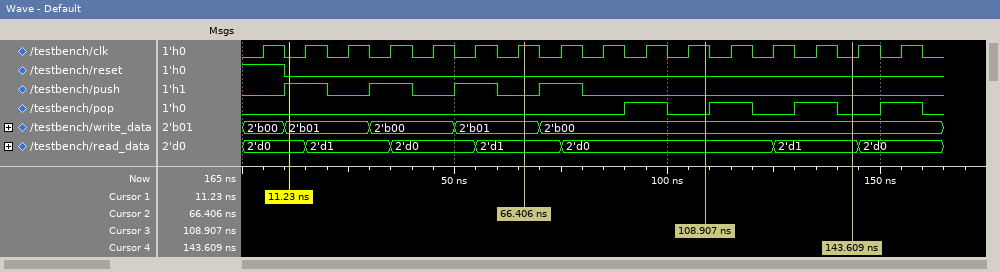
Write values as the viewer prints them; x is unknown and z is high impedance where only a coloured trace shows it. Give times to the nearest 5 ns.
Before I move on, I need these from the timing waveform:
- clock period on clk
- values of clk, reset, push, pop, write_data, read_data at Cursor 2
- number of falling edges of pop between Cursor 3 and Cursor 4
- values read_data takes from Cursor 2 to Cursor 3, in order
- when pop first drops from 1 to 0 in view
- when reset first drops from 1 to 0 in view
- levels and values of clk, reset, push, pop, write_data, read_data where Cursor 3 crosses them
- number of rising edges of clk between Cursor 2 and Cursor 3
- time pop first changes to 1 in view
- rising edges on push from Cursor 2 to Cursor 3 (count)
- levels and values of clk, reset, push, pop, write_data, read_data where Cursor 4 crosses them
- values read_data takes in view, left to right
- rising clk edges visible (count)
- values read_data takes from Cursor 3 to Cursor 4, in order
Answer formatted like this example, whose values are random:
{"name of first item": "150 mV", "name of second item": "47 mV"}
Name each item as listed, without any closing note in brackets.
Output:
{"clock period on clk": "10 ns", "values of clk, reset, push, pop, write_data, read_data at Cursor 2": "clk=1, reset=0, push=0, pop=0, write_data=2'b01, read_data=2'd1", "number of falling edges of pop between Cursor 3 and Cursor 4": "2", "values read_data takes from Cursor 2 to Cursor 3, in order": "2'd1, 2'd0", "when pop first drops from 1 to 0 in view": "100 ns", "when reset first drops from 1 to 0 in view": "10 ns", "levels and values of clk, reset, push, pop, write_data, read_data where Cursor 3 crosses them": "clk=1, reset=0, push=0, pop=0, write_data=2'b00, read_data=2'd0", "number of rising edges of clk between Cursor 2 and Cursor 3": "4", "time pop first changes to 1 in view": "90 ns", "rising edges on push from Cursor 2 to Cursor 3": "1", "levels and values of clk, reset, push, pop, write_data, read_data where Cursor 4 crosses them": "clk=0, reset=0, push=0, pop=0, write_data=2'b00, read_data=2'd1", "values read_data takes in view, left to right": "2'd0, 2'd1, 2'd0, 2'd1, 2'd0, 2'd1, 2'd0", "rising clk edges visible": "16", "values read_data takes from Cursor 3 to Cursor 4, in order": "2'd0, 2'd1"}
